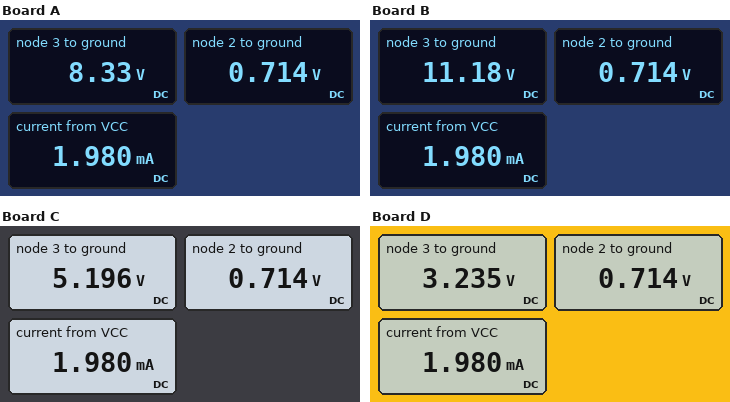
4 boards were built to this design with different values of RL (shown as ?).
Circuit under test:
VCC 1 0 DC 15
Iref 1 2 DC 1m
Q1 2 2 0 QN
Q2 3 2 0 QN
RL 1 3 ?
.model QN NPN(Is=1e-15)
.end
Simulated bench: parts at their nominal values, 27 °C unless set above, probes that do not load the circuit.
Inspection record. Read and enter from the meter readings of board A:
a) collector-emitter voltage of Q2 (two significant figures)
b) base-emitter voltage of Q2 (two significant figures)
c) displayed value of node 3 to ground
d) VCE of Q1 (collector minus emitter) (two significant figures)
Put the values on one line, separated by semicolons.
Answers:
8.3 V; 710 mV; 8.33 V; 710 mV
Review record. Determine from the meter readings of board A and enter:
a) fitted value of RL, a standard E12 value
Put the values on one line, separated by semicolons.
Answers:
6.8 kΩ
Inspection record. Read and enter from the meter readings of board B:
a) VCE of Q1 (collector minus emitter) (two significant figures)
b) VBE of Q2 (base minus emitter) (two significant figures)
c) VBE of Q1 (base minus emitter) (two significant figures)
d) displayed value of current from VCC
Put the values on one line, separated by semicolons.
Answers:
710 mV; 710 mV; 710 mV; 1.980 mA
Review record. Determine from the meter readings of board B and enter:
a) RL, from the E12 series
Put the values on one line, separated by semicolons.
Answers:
3.9 kΩ
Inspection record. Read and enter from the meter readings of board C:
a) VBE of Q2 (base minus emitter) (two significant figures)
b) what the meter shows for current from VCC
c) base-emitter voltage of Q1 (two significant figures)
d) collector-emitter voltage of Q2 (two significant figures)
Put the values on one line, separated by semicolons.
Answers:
710 mV; 1.980 mA; 710 mV; 5.2 V
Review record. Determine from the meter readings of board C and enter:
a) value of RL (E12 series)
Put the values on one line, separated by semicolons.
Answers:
10 kΩ
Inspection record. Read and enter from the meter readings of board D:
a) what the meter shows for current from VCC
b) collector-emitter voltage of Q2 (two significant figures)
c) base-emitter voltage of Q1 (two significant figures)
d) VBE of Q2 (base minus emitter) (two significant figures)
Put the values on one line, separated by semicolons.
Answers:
1.980 mA; 3.2 V; 710 mV; 710 mV
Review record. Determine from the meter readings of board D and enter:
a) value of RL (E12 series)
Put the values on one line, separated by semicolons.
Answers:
12 kΩ
